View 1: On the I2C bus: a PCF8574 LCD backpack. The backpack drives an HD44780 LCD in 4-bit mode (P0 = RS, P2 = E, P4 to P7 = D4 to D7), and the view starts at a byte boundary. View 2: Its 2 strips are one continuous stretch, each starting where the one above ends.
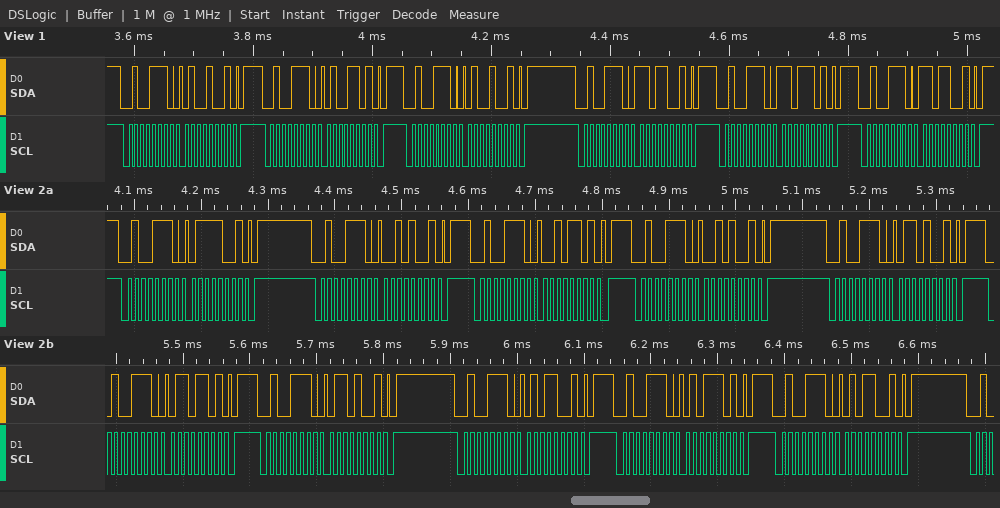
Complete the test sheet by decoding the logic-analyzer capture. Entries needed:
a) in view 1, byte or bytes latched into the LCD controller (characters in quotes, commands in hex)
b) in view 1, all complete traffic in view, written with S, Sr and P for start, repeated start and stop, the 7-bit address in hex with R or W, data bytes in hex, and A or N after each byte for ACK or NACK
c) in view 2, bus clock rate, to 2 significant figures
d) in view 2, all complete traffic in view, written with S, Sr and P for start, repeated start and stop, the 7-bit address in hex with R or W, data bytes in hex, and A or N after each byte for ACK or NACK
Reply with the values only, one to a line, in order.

'M'
S 27W A 49 A P S 27W A 4D A P S 27W A 49 A P S 27W A D9 A P S 27W A DD A P S 27W A D9 A P
100 kHz
S 27W A 79 A P S 27W A 29 A P S 27W A 2D A P S 27W A 29 A P S 27W A 69 A P S 27W A 6D A P S 27W A 69 A P S 27W A 59 A P S 27W A 5D A P S 27W A 59 A P
